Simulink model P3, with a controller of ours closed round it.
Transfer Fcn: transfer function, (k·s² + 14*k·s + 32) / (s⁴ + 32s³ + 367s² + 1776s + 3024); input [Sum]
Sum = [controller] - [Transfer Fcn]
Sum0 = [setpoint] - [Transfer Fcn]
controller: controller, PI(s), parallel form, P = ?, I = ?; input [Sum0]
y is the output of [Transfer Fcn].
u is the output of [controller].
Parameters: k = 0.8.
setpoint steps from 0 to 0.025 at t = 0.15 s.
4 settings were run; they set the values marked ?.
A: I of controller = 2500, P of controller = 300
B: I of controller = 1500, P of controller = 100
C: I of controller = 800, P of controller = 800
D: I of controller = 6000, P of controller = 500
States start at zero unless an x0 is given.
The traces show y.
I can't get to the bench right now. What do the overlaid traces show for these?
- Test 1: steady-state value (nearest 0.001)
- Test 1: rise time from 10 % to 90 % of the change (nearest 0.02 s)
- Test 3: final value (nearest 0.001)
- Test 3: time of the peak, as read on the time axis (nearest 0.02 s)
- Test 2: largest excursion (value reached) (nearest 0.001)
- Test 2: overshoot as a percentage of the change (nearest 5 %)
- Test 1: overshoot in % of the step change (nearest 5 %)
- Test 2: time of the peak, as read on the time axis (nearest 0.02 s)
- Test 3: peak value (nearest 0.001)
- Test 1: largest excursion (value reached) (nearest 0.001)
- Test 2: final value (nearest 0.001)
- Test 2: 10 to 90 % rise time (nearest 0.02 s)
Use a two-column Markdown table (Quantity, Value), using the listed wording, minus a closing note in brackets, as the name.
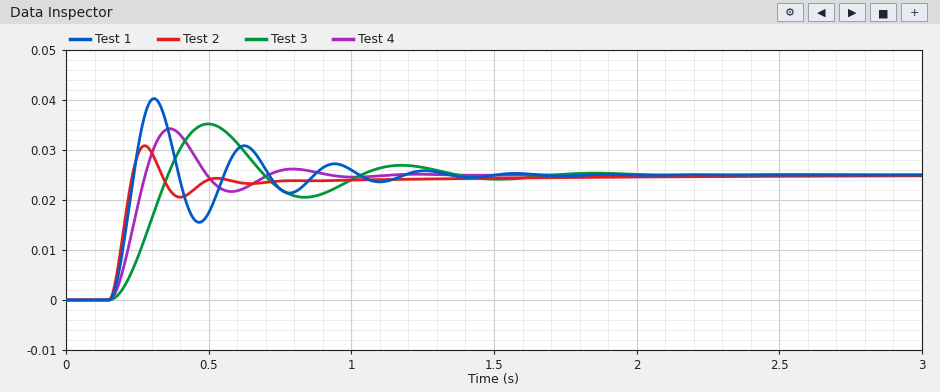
| Quantity | Value |
|---|---|
| Test 1: steady-state value | 0.025 |
| Test 1: rise time from 10 % to 90 % of the change | 0.06 s |
| Test 3: final value | 0.025 |
| Test 3: time of the peak, as read on the time axis | 0.50 s |
| Test 2: largest excursion (value reached) | 0.031 |
| Test 2: overshoot as a percentage of the change | 25 % |
| Test 1: overshoot in % of the step change | 60 % |
| Test 2: time of the peak, as read on the time axis | 0.28 s |
| Test 3: peak value | 0.035 |
| Test 1: largest excursion (value reached) | 0.040 |
| Test 2: final value | 0.025 |
| Test 2: 10 to 90 % rise time | 0.06 s |
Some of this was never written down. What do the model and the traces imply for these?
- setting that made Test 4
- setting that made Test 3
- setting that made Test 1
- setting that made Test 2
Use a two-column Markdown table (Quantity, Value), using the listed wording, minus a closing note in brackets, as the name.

| Quantity | Value |
|---|---|
| setting that made Test 4 | A |
| setting that made Test 3 | B |
| setting that made Test 1 | D |
| setting that made Test 2 | C |
